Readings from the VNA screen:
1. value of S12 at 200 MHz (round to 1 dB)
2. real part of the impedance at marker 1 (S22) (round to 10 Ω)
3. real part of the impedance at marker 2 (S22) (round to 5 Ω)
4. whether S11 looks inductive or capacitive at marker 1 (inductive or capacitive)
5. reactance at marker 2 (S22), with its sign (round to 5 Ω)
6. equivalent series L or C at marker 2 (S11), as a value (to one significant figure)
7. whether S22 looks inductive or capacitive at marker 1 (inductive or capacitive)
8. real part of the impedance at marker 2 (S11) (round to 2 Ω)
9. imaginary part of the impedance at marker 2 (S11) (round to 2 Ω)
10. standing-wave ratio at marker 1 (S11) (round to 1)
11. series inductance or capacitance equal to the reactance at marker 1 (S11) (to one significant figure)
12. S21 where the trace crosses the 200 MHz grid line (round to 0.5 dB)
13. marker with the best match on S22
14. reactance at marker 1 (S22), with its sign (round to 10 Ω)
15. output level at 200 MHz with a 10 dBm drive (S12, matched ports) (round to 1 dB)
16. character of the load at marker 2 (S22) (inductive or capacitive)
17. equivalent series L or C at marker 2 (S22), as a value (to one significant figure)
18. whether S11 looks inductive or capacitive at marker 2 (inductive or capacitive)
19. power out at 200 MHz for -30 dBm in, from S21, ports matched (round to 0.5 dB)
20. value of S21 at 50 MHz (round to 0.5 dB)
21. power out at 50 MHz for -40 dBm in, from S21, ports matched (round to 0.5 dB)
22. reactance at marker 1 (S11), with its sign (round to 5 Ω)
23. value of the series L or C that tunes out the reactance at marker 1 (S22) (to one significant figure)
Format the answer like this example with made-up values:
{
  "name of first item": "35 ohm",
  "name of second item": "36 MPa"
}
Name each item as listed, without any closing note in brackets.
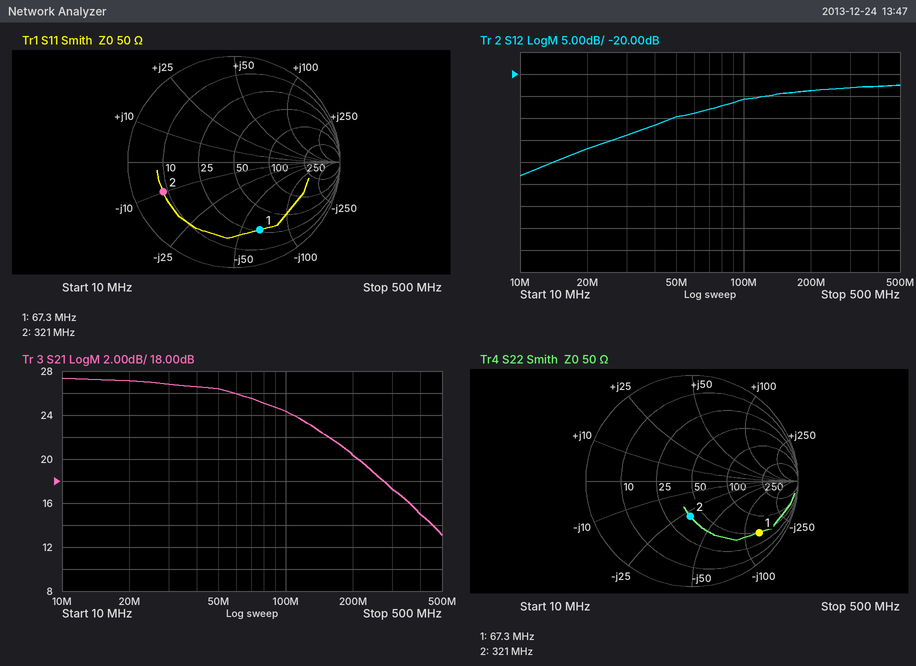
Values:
{
  "value of S12 at 200 MHz": "-24 dB",
  "real part of the impedance at marker 1 (S22)": "50 Ω",
  "real part of the impedance at marker 2 (S22)": "40 Ω",
  "whether S11 looks inductive or capacitive at marker 1": "capacitive",
  "reactance at marker 2 (S22), with its sign": "-30 Ω",
  "equivalent series L or C at marker 2 (S11), as a value": "50 pF",
  "whether S22 looks inductive or capacitive at marker 1": "capacitive",
  "real part of the impedance at marker 2 (S11)": "8 Ω",
  "imaginary part of the impedance at marker 2 (S11)": "-10 Ω",
  "standing-wave ratio at marker 1 (S11)": "5",
  "series inductance or capacitance equal to the reactance at marker 1 (S11)": "40 pF",
  "S21 where the trace crosses the 200 MHz grid line": "20.5 dB",
  "marker with the best match on S22": "marker 2",
  "reactance at marker 1 (S22), with its sign": "-130 Ω",
  "output level at 200 MHz with a 10 dBm drive (S12, matched ports)": "-14 dBm",
  "character of the load at marker 2 (S22)": "capacitive",
  "equivalent series L or C at marker 2 (S22), as a value": "20 pF",
  "whether S11 looks inductive or capacitive at marker 2": "capacitive",
  "power out at 200 MHz for -30 dBm in, from S21, ports matched": "-9.5 dBm",
  "value of S21 at 50 MHz": "26.5 dB",
  "power out at 50 MHz for -40 dBm in, from S21, ports matched": "-13.5 dBm",
  "reactance at marker 1 (S11), with its sign": "-65 Ω",
  "value of the series L or C that tunes out the reactance at marker 1 (S22)": "300 nH"
}
